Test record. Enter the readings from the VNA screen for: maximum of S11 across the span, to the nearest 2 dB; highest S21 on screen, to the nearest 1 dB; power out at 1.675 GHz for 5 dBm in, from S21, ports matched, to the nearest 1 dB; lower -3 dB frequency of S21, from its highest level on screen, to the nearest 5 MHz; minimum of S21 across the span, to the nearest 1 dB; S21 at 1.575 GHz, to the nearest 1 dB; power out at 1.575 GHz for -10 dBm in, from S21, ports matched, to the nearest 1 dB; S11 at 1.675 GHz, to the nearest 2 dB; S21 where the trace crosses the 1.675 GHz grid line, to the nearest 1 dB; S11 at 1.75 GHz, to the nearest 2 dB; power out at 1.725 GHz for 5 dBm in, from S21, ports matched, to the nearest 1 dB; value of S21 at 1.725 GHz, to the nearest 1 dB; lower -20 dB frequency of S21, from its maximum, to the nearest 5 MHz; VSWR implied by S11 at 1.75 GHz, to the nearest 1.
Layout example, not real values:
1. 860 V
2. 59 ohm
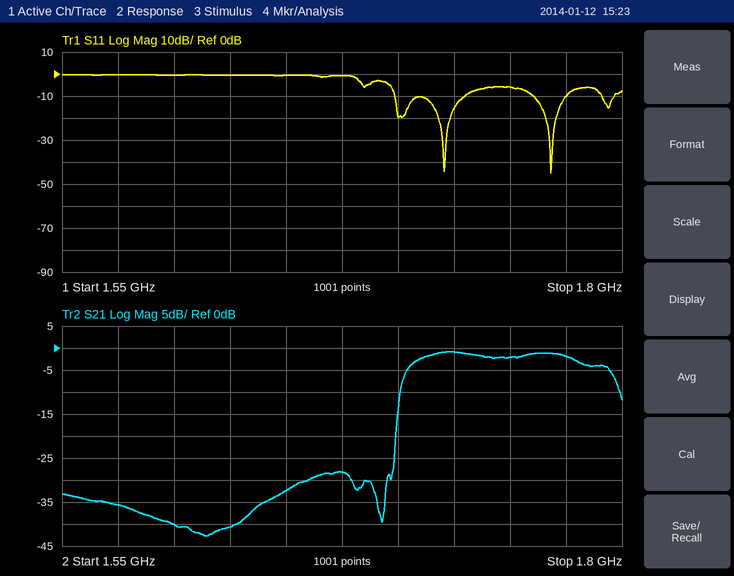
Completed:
1. 0 dB
2. -1 dB
3. -23 dBm
4. 1.705 GHz
5. -43 dB
6. -36 dB
7. -46 dBm
8. 0 dB
9. -28 dB
10. -6 dB
11. 4 dBm
12. -1 dB
13. 1.700 GHz
14. 3
